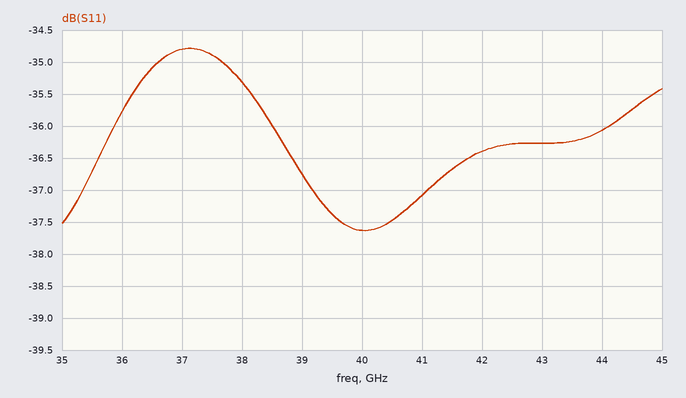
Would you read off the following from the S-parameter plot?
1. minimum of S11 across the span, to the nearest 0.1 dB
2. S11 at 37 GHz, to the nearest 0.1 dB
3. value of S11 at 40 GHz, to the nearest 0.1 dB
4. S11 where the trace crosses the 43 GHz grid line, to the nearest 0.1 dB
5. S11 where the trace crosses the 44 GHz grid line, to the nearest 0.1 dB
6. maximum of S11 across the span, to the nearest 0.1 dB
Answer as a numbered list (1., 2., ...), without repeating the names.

1. -37.6 dB
2. -34.8 dB
3. -37.6 dB
4. -36.3 dB
5. -36.1 dB
6. -34.8 dB
